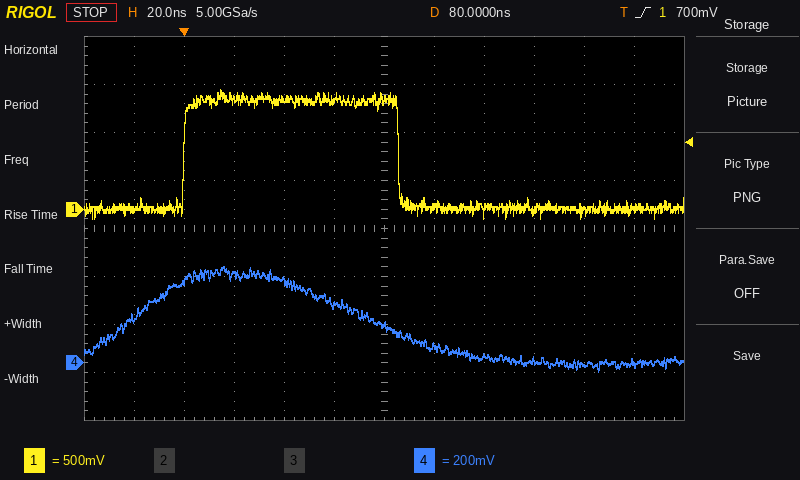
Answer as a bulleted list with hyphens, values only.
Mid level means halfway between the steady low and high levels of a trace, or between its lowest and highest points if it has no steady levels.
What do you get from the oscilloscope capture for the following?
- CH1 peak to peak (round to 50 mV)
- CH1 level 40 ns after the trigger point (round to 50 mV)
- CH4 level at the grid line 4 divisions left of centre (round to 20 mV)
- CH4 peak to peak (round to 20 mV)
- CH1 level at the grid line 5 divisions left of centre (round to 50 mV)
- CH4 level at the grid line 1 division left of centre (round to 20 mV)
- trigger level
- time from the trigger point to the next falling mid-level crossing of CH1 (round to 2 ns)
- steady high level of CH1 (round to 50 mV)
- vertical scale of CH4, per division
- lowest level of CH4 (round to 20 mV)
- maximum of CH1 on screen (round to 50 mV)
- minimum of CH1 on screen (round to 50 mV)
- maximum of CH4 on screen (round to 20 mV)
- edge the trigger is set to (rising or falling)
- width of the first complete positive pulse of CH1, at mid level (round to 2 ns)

- 1.35 V
- 1.15 V
- 340 mV
- 440 mV
- 0 mV
- 240 mV
- 700 mV
- 86 ns
- 1.15 V
- 200 mV
- -40 mV
- 1.25 V
- -100 mV
- 400 mV
- rising
- 86 ns
